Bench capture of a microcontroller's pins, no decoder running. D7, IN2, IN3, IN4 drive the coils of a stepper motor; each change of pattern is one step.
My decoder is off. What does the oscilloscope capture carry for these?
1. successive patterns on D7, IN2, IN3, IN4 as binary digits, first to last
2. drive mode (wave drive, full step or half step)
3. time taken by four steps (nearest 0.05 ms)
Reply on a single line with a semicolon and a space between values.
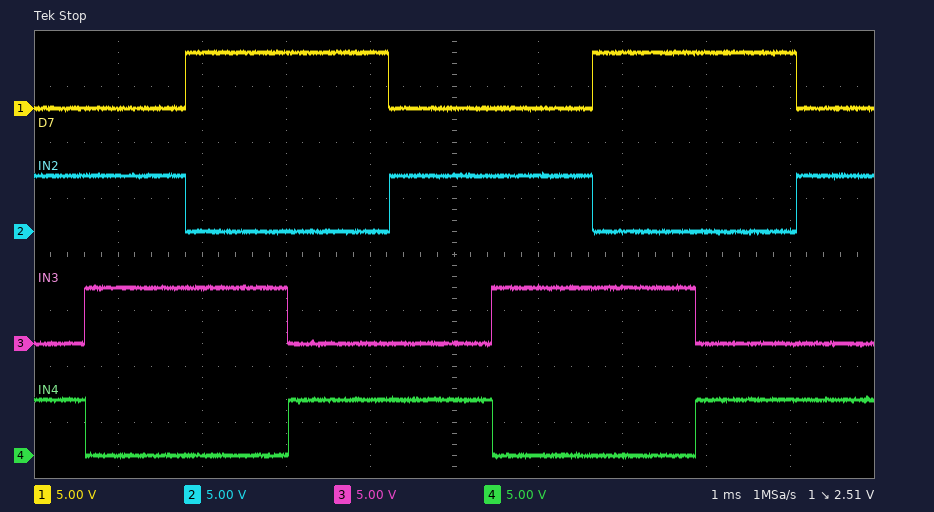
0101 0110 1010 1001 0101 0110 1010 1001 0101; full step; 4.85 ms
